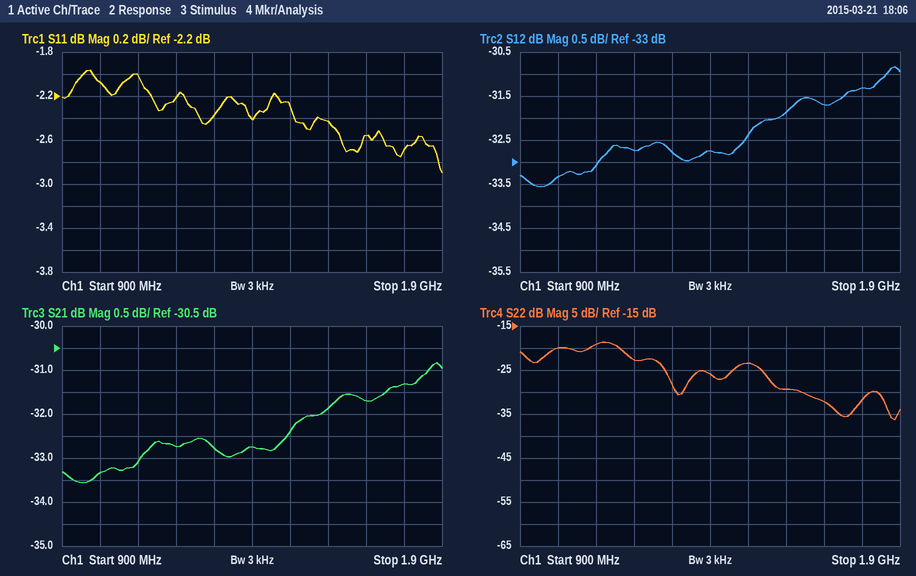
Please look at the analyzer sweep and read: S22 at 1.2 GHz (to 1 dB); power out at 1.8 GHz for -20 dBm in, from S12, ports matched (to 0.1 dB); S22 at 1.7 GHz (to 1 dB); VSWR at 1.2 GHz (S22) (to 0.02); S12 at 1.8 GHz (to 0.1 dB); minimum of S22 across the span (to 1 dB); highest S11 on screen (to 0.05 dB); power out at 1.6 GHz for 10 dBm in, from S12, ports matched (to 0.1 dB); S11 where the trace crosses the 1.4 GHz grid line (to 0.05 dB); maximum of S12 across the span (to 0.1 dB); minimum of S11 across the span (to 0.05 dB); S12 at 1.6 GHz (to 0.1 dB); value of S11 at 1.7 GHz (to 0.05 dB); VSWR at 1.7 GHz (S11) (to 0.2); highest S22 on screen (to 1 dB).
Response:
-23 dB
-51.3 dBm
-32 dB
1.16
-31.3 dB
-36 dB
-1.95 dB
-21.9 dBm
-2.40 dB
-30.8 dB
-2.90 dB
-31.9 dB
-2.55 dB
6.8
-19 dB
